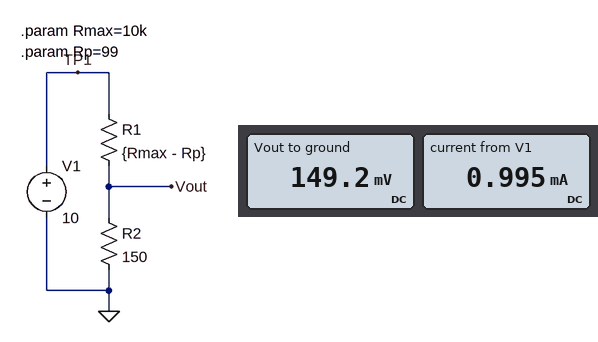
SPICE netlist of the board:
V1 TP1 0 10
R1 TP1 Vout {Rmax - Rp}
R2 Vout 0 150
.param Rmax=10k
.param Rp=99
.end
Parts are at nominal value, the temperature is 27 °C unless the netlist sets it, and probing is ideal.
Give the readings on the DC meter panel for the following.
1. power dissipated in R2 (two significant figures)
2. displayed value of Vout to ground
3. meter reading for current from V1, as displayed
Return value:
150 µW
149.2 mV
0.995 mA
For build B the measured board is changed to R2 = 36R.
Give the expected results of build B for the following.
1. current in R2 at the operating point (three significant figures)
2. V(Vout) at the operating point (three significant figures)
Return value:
1.01 mA
36.2 mV
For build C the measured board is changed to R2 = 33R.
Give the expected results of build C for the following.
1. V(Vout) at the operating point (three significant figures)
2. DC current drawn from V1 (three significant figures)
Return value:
33.2 mV
1.01 mA
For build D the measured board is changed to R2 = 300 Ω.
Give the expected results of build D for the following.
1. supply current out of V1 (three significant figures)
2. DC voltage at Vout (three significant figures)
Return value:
980 µA
294 mV
